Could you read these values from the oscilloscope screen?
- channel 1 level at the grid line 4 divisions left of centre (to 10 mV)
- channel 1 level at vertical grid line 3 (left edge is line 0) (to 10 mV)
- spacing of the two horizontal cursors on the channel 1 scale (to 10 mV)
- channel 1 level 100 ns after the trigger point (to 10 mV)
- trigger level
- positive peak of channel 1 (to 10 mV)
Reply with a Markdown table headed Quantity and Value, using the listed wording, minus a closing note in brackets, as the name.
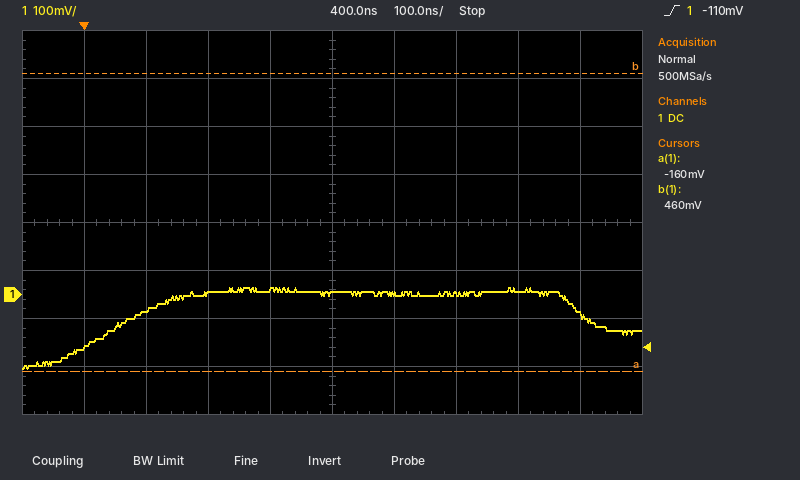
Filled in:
| Quantity | Value |
|---|---|
| channel 1 level at the grid line 4 divisions left of centre | -110 mV |
| channel 1 level at vertical grid line 3 (left edge is line 0) | 0 mV |
| spacing of the two horizontal cursors on the channel 1 scale | 620 mV |
| channel 1 level 100 ns after the trigger point | -30 mV |
| trigger level | -110 mV |
| positive peak of channel 1 | 10 mV |
